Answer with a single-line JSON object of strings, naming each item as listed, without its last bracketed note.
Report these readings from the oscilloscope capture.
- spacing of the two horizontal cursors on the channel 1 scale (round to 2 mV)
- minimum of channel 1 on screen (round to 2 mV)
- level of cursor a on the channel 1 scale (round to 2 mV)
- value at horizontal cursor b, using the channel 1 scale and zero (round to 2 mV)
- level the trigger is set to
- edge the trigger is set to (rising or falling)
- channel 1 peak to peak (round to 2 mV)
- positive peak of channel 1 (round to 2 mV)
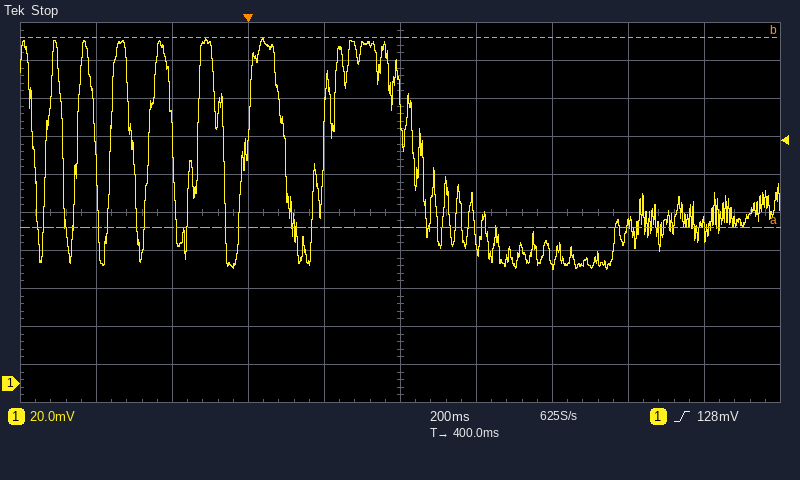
{"spacing of the two horizontal cursors on the channel 1 scale": "100 mV", "minimum of channel 1 on screen": "60 mV", "level of cursor a on the channel 1 scale": "82 mV", "value at horizontal cursor b, using the channel 1 scale and zero": "182 mV", "level the trigger is set to": "128 mV", "edge the trigger is set to": "rising", "channel 1 peak to peak": "122 mV", "positive peak of channel 1": "182 mV"}
